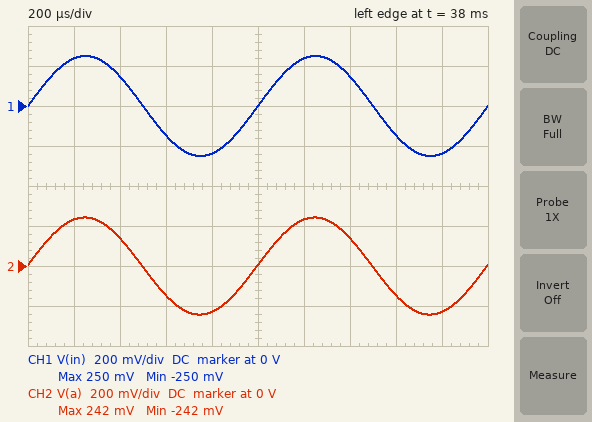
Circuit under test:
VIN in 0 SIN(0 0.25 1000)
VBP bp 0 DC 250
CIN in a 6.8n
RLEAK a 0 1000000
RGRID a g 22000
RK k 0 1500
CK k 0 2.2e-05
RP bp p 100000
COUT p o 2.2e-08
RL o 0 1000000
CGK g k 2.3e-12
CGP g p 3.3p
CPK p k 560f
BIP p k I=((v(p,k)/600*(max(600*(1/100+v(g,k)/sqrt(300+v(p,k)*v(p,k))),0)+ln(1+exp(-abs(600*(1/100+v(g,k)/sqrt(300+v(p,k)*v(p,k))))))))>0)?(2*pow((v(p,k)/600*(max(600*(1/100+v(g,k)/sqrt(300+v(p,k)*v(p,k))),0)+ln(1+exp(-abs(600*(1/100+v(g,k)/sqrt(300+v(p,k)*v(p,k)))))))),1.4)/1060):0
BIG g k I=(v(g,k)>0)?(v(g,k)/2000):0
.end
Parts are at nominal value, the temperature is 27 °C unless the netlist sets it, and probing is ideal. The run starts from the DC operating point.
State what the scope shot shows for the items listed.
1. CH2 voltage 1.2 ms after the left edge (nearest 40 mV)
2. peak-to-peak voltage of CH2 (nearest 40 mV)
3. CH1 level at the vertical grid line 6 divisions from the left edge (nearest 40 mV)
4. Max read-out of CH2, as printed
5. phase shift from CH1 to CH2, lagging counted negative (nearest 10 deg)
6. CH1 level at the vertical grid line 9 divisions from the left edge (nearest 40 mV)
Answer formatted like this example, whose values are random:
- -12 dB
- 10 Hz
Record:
- 240 mV
- 480 mV
- 240 mV
- 242 mV
- 0 deg
- -240 mV
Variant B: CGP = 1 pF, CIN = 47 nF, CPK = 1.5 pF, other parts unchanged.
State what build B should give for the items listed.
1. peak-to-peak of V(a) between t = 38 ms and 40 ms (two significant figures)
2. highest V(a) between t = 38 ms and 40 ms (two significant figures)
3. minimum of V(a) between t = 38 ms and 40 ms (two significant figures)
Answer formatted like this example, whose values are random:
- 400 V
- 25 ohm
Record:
- 500 mV
- 250 mV
- -250 mV
